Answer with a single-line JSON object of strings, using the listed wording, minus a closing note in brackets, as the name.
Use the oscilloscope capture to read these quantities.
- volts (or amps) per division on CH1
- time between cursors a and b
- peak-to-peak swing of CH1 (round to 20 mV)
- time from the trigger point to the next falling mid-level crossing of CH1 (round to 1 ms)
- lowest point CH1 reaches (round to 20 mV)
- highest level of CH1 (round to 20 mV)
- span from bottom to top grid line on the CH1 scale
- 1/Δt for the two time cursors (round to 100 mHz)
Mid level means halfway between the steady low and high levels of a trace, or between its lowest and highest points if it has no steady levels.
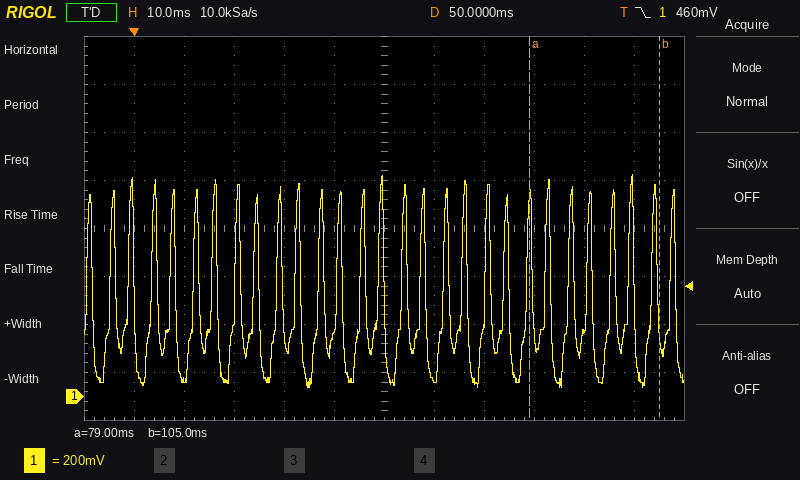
{"volts (or amps) per division on CH1": "200 mV", "time between cursors a and b": "26 ms", "peak-to-peak swing of CH1": "880 mV", "time from the trigger point to the next falling mid-level crossing of CH1": "5 ms", "lowest point CH1 reaches": "40 mV", "highest level of CH1": "920 mV", "span from bottom to top grid line on the CH1 scale": "1.6 V", "1/Δt for the two time cursors": "38.5 Hz"}
